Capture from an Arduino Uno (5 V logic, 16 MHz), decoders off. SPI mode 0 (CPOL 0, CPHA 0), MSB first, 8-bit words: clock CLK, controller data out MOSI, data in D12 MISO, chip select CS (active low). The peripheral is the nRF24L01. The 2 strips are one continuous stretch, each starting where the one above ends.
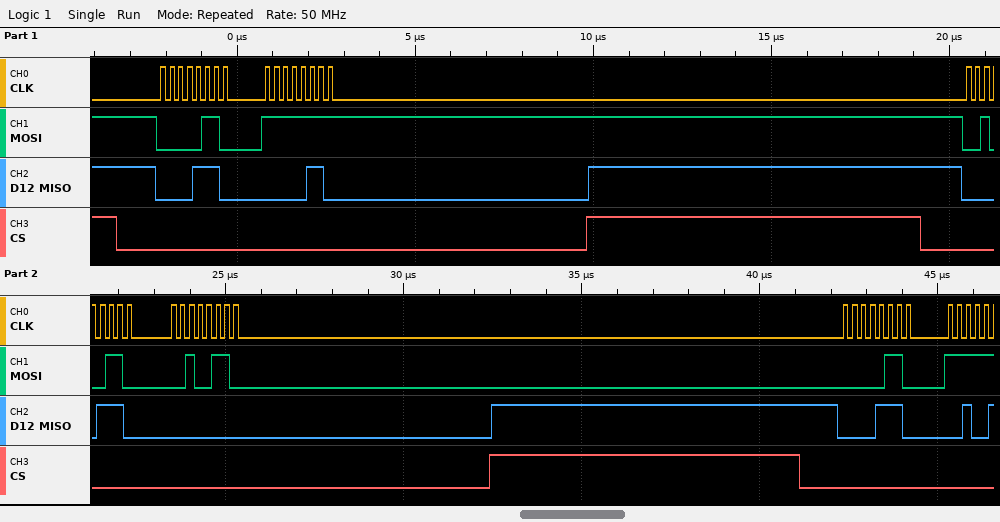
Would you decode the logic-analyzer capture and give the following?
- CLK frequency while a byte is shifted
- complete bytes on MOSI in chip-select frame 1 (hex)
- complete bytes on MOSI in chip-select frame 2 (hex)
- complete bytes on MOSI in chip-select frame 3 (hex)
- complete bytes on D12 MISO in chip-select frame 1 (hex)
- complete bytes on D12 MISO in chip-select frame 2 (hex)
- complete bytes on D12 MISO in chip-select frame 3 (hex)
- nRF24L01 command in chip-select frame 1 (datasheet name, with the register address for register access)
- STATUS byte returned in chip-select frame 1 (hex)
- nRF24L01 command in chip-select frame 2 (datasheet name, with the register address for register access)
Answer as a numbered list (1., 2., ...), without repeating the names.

1. 4 MHz
2. 06 FF
3. 26 26
4. 06
5. 0E 06
6. 0E 00
7. 0E
8. R_REGISTER 0x06
9. 0x0E
10. W_REGISTER 0x06
